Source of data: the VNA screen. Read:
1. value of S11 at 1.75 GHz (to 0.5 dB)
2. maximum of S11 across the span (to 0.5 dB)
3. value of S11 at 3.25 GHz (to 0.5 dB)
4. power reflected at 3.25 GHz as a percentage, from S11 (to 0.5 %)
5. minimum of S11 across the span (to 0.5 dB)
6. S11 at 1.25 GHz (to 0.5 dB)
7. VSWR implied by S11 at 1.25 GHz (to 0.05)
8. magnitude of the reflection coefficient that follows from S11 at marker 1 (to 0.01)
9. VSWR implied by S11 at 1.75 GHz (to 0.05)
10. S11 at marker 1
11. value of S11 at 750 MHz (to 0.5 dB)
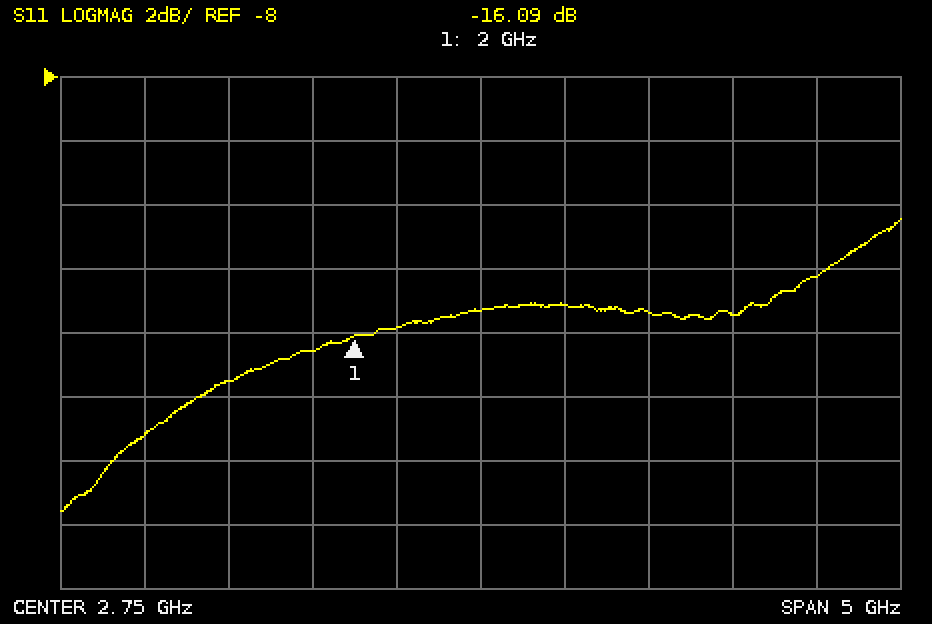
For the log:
-16.5 dB
-12.5 dB
-15.0 dB
3.0 %
-21.5 dB
-17.5 dB
1.30
0.16
1.35
-16.09 dB
-19.0 dB
